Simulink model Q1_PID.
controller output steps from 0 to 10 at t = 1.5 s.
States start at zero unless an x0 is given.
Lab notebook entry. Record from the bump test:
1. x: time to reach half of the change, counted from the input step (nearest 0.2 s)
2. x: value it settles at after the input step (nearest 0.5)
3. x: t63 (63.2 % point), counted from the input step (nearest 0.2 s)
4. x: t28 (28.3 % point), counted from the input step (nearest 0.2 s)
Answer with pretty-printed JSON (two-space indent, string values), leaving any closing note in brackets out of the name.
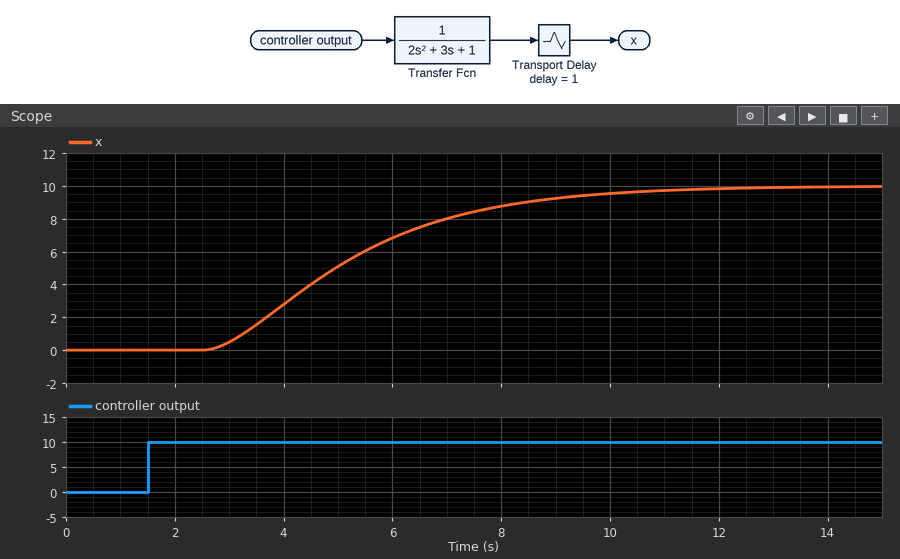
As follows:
{
  "x: time to reach half of the change, counted from the input step": "3.4 s",
  "x: value it settles at after the input step": "10.0",
  "x: t63 (63.2 % point), counted from the input step": "4.2 s",
  "x: t28 (28.3 % point), counted from the input step": "2.6 s"
}
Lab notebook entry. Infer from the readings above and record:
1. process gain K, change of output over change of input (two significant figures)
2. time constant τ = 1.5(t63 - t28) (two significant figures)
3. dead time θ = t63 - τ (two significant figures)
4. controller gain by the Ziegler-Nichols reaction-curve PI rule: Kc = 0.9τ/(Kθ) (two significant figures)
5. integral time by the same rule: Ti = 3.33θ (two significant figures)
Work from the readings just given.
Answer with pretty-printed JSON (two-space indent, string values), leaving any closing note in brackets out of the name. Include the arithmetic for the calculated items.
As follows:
{
  "process gain K, change of output over change of input": "(10 - 0) / 10 = 1.0",
  "time constant τ = 1.5(t63 - t28)": "1.5 × (4.2 - 2.6) = 2.4 s",
  "dead time θ = t63 - τ": "4.2 - 2.4 = 1.8 s",
  "controller gain by the Ziegler-Nichols reaction-curve PI rule: Kc = 0.9τ/(Kθ)": "0.9 × 2.4 / (1 × 1.8) = 1.2",
  "integral time by the same rule: Ti = 3.33θ": "3.33 × 1.8 = 6.0 s"
}
